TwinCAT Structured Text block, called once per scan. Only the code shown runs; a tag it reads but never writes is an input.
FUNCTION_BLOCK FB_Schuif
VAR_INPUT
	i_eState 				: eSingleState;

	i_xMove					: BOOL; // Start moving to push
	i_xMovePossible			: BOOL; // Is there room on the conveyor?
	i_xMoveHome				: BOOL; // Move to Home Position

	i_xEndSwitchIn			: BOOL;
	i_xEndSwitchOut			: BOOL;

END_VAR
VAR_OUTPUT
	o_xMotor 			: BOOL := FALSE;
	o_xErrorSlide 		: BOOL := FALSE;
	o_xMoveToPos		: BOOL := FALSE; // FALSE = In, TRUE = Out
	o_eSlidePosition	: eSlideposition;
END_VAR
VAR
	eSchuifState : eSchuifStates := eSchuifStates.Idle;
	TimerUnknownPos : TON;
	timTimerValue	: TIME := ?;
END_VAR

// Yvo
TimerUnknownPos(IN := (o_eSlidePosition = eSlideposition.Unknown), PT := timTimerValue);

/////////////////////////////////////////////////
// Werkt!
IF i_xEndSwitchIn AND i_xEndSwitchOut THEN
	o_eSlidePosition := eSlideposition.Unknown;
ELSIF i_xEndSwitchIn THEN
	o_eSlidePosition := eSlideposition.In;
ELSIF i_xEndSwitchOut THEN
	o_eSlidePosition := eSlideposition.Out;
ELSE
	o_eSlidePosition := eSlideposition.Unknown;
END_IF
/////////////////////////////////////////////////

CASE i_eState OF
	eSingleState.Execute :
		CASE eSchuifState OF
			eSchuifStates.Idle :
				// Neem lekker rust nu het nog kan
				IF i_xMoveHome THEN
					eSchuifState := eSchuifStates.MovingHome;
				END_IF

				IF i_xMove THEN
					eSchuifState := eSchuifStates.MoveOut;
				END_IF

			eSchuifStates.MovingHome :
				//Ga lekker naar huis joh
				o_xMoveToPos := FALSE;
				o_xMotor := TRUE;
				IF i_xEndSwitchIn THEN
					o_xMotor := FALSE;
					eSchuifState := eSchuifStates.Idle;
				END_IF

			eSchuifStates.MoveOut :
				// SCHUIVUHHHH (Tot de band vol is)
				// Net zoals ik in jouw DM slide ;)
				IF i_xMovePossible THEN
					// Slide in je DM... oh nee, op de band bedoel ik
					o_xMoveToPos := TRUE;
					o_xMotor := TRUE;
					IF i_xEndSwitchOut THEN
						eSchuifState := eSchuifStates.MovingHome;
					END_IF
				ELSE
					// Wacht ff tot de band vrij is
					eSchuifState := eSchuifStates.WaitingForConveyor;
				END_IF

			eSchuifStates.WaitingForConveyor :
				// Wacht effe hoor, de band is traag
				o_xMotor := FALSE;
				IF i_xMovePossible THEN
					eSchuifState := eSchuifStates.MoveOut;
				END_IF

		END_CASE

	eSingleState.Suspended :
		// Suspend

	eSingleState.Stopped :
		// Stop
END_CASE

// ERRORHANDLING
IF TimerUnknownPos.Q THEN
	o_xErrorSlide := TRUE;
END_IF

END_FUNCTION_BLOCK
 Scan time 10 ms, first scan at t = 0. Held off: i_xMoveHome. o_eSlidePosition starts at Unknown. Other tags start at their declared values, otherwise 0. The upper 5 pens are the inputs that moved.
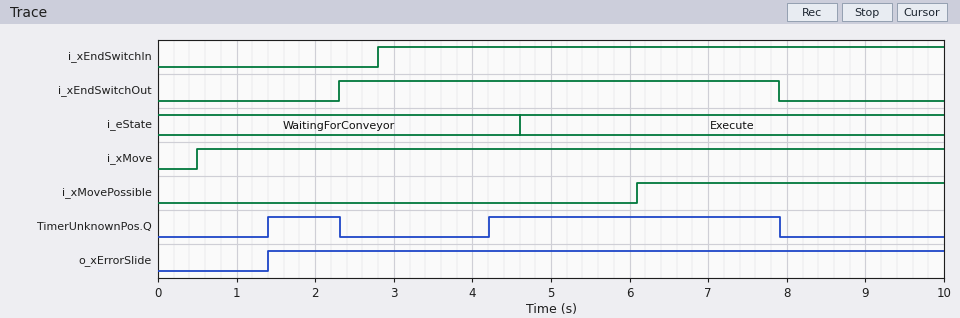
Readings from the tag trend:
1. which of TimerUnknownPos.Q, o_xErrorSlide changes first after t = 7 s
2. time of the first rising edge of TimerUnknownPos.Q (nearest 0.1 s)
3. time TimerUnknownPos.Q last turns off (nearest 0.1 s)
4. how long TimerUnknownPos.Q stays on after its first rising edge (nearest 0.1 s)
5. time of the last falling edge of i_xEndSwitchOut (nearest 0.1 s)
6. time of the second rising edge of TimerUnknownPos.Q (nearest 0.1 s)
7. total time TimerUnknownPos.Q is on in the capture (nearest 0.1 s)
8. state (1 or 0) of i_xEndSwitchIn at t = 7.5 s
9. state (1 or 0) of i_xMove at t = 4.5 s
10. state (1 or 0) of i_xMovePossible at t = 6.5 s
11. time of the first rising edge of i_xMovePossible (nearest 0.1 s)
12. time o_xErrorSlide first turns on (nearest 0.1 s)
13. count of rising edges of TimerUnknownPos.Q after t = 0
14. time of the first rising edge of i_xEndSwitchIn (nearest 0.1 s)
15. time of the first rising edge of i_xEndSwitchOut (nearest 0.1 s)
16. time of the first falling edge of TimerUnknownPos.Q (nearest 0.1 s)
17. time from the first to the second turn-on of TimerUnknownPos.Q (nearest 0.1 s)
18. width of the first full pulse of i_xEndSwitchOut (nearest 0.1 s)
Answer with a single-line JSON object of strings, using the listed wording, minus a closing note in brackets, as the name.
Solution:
{"which of TimerUnknownPos.Q, o_xErrorSlide changes first after t = 7 s": "TimerUnknownPos.Q", "time of the first rising edge of TimerUnknownPos.Q": "1.4 s", "time TimerUnknownPos.Q last turns off": "7.9 s", "how long TimerUnknownPos.Q stays on after its first rising edge": "0.9 s", "time of the last falling edge of i_xEndSwitchOut": "7.9 s", "time of the second rising edge of TimerUnknownPos.Q": "4.2 s", "total time TimerUnknownPos.Q is on in the capture": "4.6 s", "state (1 or 0) of i_xEndSwitchIn at t = 7.5 s": "1", "state (1 or 0) of i_xMove at t = 4.5 s": "1", "state (1 or 0) of i_xMovePossible at t = 6.5 s": "1", "time of the first rising edge of i_xMovePossible": "6.1 s", "time o_xErrorSlide first turns on": "1.4 s", "count of rising edges of TimerUnknownPos.Q after t = 0": "2", "time of the first rising edge of i_xEndSwitchIn": "2.8 s", "time of the first rising edge of i_xEndSwitchOut": "2.3 s", "time of the first falling edge of TimerUnknownPos.Q": "2.3 s", "time from the first to the second turn-on of TimerUnknownPos.Q": "2.8 s", "width of the first full pulse of i_xEndSwitchOut": "5.6 s"}
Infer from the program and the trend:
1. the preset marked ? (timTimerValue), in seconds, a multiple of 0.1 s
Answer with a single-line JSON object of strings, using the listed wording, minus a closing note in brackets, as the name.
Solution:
{"the preset marked ? (timTimerValue), in seconds, a multiple of 0.1 s": "1.4 s"}
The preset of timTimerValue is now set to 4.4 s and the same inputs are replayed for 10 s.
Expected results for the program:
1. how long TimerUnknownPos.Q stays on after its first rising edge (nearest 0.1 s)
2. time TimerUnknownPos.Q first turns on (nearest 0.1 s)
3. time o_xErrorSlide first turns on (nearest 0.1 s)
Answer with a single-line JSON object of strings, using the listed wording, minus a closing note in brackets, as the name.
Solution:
{"how long TimerUnknownPos.Q stays on after its first rising edge": "0.7 s", "time TimerUnknownPos.Q first turns on": "7.2 s", "time o_xErrorSlide first turns on": "7.2 s"}
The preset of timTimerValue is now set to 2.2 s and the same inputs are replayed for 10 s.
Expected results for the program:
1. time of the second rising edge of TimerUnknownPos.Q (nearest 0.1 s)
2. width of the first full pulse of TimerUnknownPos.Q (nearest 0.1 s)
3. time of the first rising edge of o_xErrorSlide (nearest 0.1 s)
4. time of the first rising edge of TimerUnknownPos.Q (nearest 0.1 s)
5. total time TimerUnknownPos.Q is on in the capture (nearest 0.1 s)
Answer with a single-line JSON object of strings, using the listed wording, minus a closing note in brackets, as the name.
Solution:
{"time of the second rising edge of TimerUnknownPos.Q": "5.0 s", "width of the first full pulse of TimerUnknownPos.Q": "0.1 s", "time of the first rising edge of o_xErrorSlide": "2.2 s", "time of the first rising edge of TimerUnknownPos.Q": "2.2 s", "total time TimerUnknownPos.Q is on in the capture": "3.0 s"}
